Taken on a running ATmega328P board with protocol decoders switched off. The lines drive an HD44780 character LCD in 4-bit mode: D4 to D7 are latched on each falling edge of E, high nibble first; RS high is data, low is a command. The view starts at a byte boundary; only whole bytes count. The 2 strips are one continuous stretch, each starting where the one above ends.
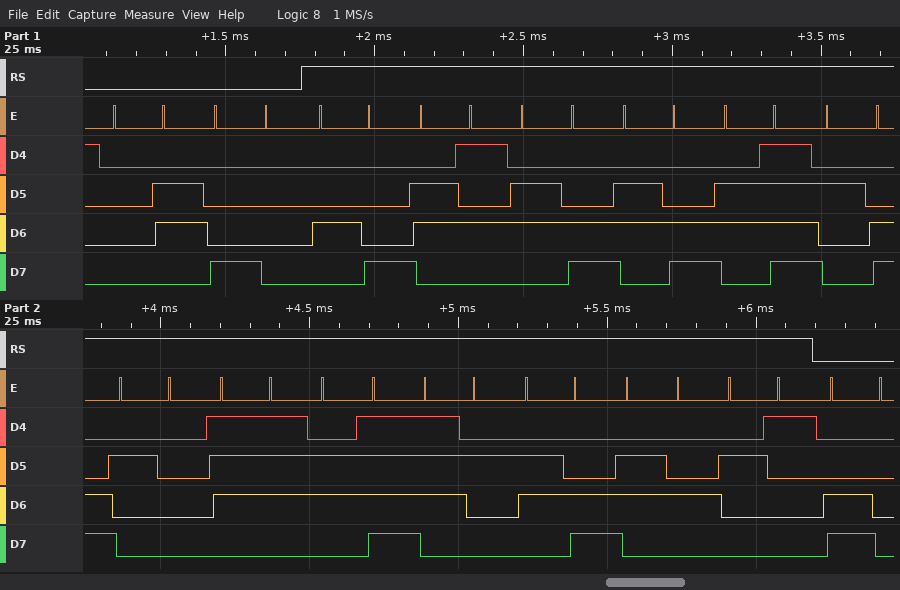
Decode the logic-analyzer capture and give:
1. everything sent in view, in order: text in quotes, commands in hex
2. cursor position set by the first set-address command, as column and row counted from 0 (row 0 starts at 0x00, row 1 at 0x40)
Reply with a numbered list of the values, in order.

1. 0x06 0x80 "Hello, world!" 0xC0
2. column 0, row 0
